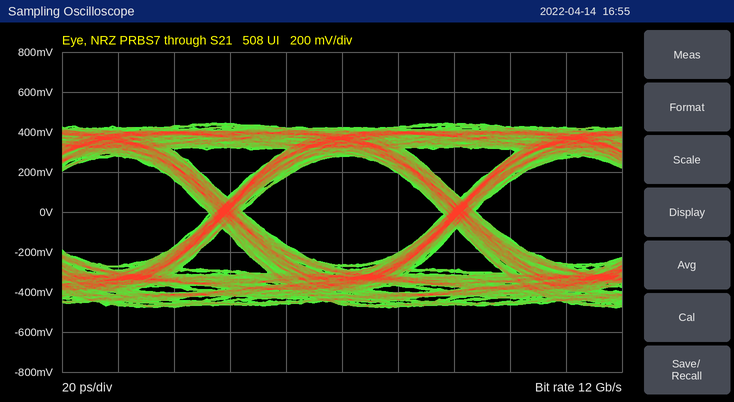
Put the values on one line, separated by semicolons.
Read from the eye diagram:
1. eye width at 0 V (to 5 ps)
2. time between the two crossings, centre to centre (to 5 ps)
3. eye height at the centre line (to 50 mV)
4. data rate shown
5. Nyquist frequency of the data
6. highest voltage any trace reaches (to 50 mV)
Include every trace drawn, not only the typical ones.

70 ps; 85 ps; 550 mV; 12 Gb/s; 6 GHz; 450 mV
